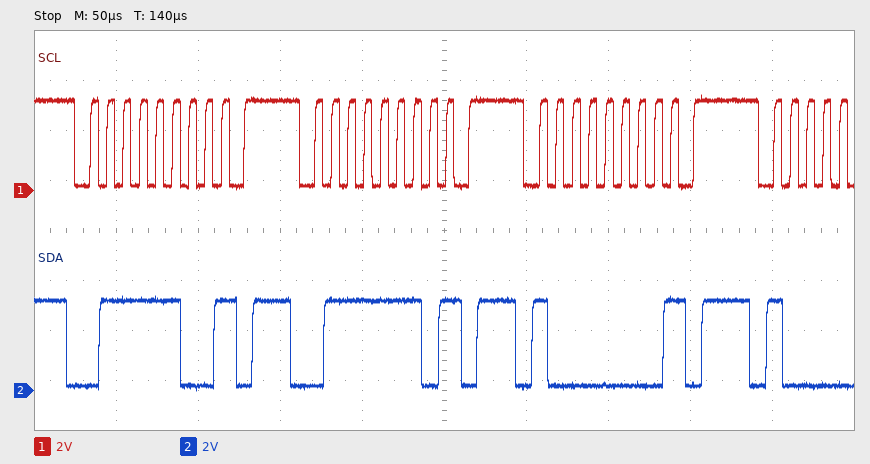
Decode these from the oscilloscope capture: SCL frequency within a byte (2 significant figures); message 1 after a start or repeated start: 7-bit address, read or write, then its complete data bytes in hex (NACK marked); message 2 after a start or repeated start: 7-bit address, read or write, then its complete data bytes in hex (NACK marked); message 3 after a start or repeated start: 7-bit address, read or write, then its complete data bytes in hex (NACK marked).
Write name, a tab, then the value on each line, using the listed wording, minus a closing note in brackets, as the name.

SCL frequency within a byte	100 kHz
message 1 after a start or repeated start: 7-bit address, read or write, then its complete data bytes in hex	0x3E write NACK
message 2 after a start or repeated start: 7-bit address, read or write, then its complete data bytes in hex	0x3F write NACK
message 3 after a start or repeated start: 7-bit address, read or write, then its complete data bytes in hex	0x40 write NACK
